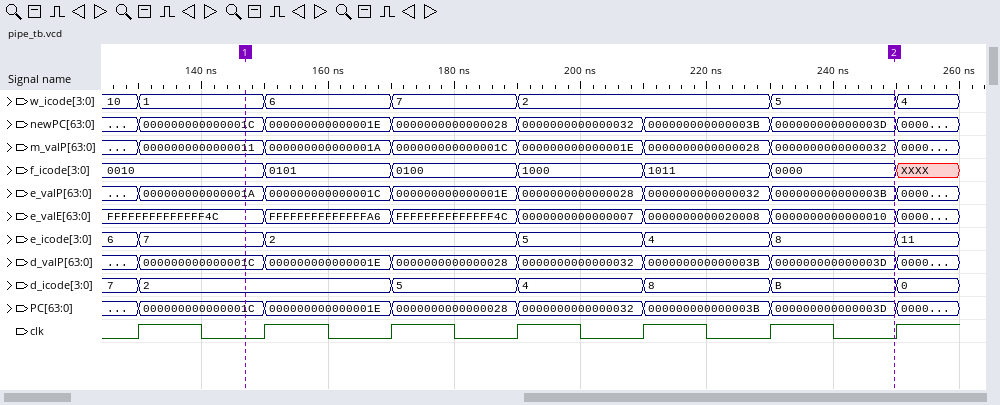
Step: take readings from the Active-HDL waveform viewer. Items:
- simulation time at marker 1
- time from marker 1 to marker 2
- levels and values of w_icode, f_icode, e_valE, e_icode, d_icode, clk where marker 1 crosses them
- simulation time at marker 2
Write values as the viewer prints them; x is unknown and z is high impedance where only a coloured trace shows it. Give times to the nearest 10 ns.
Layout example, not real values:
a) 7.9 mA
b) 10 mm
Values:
a) 150 ns
b) 100 ns
c) w_icode=1, f_icode=0010, e_valE=FFFFFFFFFFFFFF4C, e_icode=7, d_icode=2, clk=0
d) 250 ns
